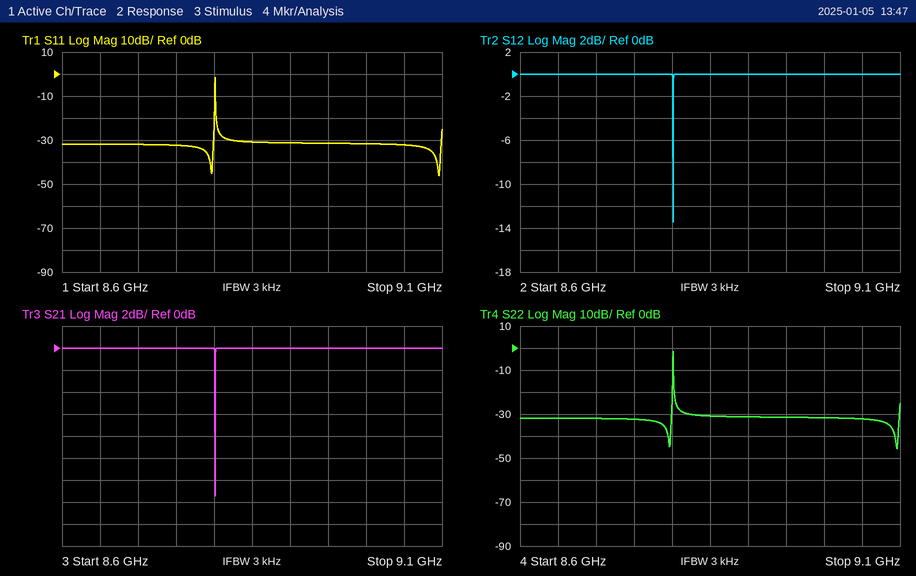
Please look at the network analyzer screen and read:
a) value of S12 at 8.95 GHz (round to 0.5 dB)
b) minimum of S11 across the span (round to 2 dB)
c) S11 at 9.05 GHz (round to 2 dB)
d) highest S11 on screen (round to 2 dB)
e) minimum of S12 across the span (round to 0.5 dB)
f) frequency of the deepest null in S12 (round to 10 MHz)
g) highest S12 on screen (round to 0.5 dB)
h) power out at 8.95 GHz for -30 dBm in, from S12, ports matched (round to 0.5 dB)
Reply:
0.0 dB
-46 dB
-32 dB
-2 dB
-13.5 dB
8.80 GHz
0.0 dB
-30.0 dBm
